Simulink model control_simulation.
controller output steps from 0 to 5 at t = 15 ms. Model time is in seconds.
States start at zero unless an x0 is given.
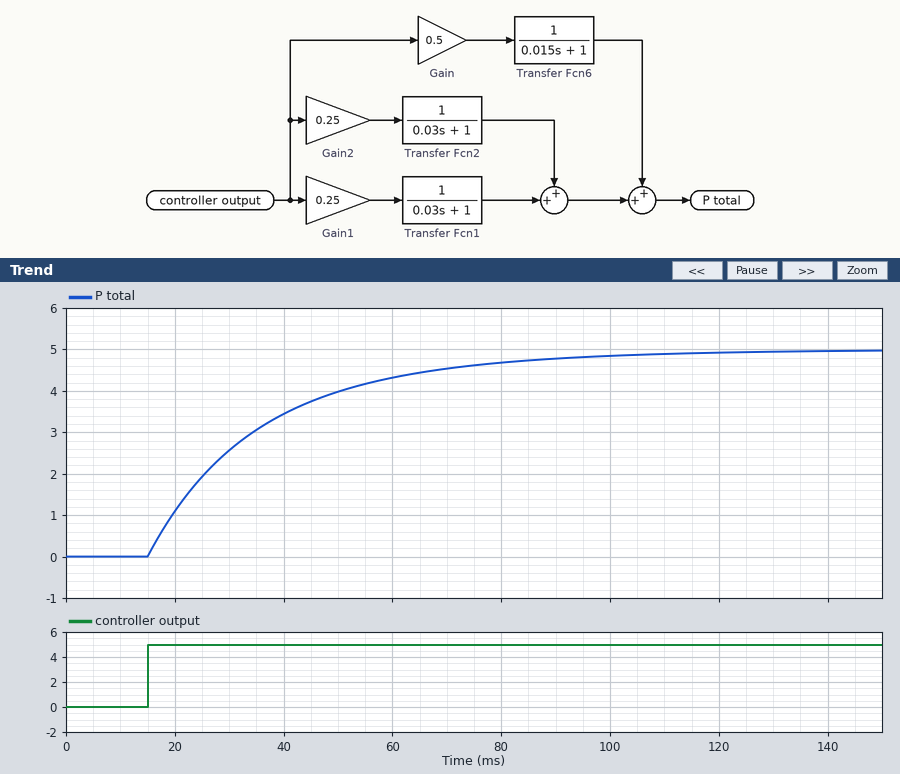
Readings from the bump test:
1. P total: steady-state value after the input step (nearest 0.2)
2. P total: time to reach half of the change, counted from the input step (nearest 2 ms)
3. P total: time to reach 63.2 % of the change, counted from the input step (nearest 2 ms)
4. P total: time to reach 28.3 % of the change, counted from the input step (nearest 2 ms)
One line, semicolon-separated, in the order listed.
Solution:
5.0; 14 ms; 22 ms; 6 ms
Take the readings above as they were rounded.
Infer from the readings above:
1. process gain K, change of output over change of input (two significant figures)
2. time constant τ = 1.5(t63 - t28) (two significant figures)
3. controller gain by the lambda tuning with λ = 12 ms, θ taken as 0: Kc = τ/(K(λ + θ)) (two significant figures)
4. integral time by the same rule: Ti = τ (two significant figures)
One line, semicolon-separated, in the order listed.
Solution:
1.0; 24 ms; 2.0; 24 ms
